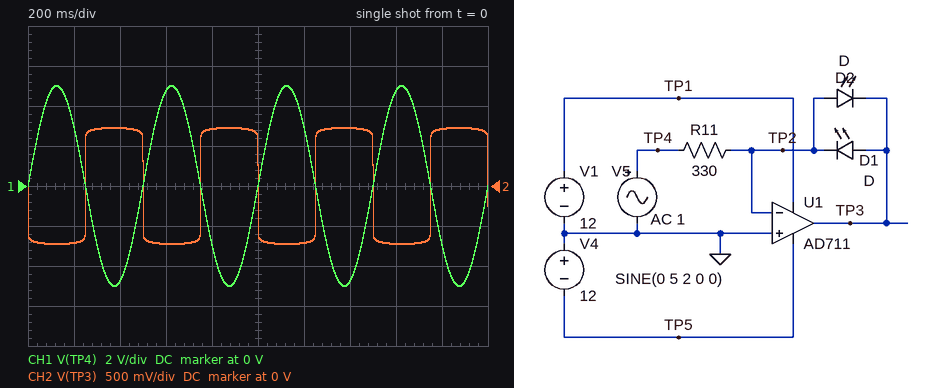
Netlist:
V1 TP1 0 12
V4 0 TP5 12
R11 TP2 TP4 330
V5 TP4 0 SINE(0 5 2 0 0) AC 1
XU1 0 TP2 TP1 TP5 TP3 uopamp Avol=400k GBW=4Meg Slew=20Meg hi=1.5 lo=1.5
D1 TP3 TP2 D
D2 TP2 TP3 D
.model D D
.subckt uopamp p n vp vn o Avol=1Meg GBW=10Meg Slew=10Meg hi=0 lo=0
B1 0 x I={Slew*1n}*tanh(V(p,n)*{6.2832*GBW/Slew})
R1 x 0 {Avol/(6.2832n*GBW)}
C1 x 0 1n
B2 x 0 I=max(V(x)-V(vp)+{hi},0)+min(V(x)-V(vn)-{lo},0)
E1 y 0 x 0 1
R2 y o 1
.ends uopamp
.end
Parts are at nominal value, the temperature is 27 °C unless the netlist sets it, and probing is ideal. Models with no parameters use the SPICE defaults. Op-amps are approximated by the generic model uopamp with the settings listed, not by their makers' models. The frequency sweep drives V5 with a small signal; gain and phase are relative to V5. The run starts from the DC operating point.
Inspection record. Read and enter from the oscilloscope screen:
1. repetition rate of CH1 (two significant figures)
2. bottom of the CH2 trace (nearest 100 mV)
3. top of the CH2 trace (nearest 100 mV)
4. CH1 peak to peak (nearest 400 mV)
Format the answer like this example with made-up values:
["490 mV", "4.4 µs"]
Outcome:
["2.0 Hz", "-700 mV", "700 mV", "10.0 V"]
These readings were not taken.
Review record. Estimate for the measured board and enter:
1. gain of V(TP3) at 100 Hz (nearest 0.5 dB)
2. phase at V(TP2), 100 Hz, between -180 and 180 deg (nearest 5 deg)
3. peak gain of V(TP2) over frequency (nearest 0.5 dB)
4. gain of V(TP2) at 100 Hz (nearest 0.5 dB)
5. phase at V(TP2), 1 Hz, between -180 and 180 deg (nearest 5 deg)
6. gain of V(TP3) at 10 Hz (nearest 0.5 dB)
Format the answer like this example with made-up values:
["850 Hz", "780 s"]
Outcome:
["92.0 dB", "0 deg", "0 dB", "0 dB", "0 deg", "109.0 dB"]
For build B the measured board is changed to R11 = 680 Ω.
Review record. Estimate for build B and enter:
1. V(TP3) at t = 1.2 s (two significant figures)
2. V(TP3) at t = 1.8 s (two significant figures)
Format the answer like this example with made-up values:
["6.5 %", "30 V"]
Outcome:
["-690 mV", "690 mV"]
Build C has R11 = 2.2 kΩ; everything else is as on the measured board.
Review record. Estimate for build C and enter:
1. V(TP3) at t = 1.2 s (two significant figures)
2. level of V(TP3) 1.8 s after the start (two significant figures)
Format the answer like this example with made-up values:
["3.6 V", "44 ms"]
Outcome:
["-660 mV", "660 mV"]
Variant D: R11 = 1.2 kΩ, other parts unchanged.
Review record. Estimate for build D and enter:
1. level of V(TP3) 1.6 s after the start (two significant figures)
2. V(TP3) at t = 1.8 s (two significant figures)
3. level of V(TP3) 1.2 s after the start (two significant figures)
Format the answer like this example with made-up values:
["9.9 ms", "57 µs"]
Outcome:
["-690 mV", "680 mV", "-680 mV"]
